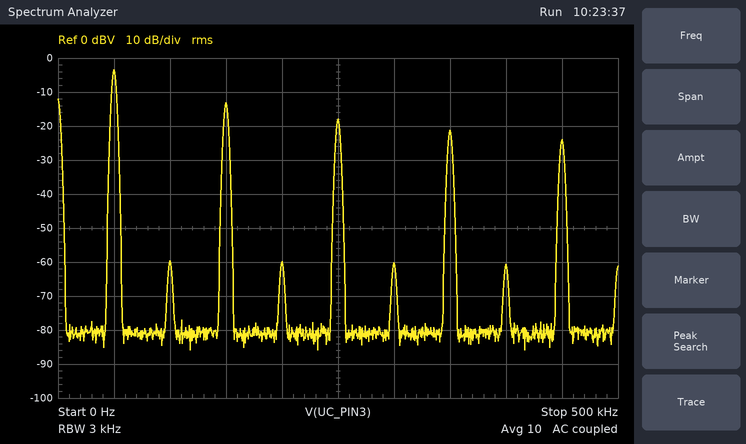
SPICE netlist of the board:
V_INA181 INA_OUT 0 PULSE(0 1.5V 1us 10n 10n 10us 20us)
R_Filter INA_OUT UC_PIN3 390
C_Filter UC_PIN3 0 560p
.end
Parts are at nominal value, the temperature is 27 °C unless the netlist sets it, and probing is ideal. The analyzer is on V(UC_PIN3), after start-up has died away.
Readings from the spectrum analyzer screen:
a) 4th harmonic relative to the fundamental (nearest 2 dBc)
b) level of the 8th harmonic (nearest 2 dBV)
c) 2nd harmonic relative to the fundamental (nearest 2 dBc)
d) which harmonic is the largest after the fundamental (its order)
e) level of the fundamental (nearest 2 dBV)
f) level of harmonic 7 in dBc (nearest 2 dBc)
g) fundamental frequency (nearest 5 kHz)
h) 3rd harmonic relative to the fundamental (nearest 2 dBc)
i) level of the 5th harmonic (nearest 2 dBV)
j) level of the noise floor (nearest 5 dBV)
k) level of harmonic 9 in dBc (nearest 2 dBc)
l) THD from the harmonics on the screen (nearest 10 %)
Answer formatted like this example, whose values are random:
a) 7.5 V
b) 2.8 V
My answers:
a) -56 dBc
b) -60 dBV
c) -56 dBc
d) 3
e) -4 dBV
f) -18 dBc
g) 50 kHz
h) -10 dBc
i) -18 dBV
j) -80 dBV
k) -20 dBc
l) 40 %
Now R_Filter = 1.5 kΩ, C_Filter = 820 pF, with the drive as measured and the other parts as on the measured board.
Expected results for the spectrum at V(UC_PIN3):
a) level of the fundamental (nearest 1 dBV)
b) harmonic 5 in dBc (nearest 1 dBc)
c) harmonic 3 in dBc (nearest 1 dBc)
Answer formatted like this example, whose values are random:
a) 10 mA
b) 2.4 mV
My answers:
a) -4 dBV
b) -20 dBc
c) -13 dBc
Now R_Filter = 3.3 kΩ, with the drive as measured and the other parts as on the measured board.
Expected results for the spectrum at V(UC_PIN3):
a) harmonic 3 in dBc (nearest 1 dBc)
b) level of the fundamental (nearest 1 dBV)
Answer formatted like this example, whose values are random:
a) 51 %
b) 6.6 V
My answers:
a) -14 dBc
b) -5 dBV
